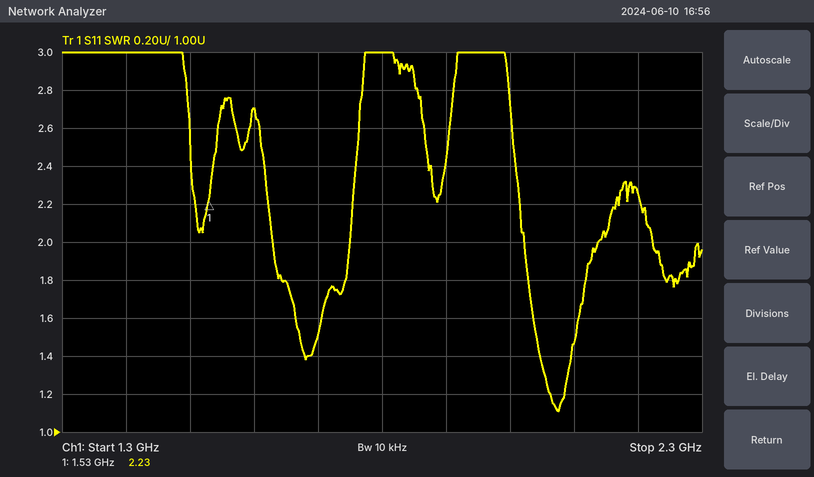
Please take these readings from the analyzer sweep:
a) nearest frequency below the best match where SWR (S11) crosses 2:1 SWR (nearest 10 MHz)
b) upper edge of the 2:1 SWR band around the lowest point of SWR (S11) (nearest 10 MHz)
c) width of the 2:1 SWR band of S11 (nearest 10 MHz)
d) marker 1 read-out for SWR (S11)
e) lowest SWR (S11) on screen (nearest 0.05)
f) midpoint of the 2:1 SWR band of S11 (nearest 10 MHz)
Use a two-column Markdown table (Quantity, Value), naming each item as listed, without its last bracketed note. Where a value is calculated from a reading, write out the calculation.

| Quantity | Value |
|---|---|
| nearest frequency below the best match where SWR (S11) crosses 2:1 SWR | 2.02 GHz |
| upper edge of the 2:1 SWR band around the lowest point of SWR (S11) | 2.14 GHz |
| width of the 2:1 SWR band of S11 | 2.14 GHz − 2.02 GHz = 120 MHz |
| marker 1 read-out for SWR | 2.23 |
| lowest SWR (S11) on screen | 1.10 |
| midpoint of the 2:1 SWR band of S11 | 2.08 GHz |
